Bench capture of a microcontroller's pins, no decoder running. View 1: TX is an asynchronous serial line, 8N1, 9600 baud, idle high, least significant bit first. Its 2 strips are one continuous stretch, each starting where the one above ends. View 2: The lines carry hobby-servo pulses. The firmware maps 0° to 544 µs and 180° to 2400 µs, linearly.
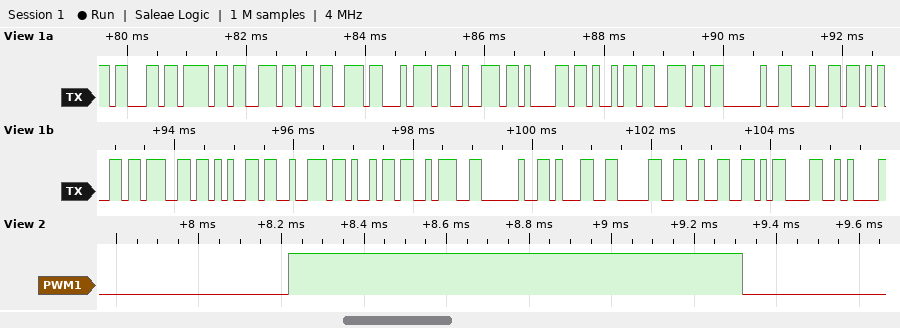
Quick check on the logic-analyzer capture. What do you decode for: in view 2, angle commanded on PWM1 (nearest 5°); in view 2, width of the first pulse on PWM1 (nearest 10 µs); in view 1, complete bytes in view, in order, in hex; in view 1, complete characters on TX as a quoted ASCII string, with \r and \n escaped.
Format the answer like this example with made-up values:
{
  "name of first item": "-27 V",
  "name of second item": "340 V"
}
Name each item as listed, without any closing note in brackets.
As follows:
{
  "in view 2, angle commanded on PWM1": "55°",
  "in view 2, width of the first pulse on PWM1": "1100 µs",
  "in view 1, complete bytes in view, in order, in hex": "63 6F 6E 73 74 72 61 69 6E 20 64 65 67 65 72 69 3A 20 31 30 32 0D 0A",
  "in view 1, complete characters on TX as a quoted ASCII string, with \\r and \\n escaped": "\"constrain degeri: 102\\r\\n\""
}
